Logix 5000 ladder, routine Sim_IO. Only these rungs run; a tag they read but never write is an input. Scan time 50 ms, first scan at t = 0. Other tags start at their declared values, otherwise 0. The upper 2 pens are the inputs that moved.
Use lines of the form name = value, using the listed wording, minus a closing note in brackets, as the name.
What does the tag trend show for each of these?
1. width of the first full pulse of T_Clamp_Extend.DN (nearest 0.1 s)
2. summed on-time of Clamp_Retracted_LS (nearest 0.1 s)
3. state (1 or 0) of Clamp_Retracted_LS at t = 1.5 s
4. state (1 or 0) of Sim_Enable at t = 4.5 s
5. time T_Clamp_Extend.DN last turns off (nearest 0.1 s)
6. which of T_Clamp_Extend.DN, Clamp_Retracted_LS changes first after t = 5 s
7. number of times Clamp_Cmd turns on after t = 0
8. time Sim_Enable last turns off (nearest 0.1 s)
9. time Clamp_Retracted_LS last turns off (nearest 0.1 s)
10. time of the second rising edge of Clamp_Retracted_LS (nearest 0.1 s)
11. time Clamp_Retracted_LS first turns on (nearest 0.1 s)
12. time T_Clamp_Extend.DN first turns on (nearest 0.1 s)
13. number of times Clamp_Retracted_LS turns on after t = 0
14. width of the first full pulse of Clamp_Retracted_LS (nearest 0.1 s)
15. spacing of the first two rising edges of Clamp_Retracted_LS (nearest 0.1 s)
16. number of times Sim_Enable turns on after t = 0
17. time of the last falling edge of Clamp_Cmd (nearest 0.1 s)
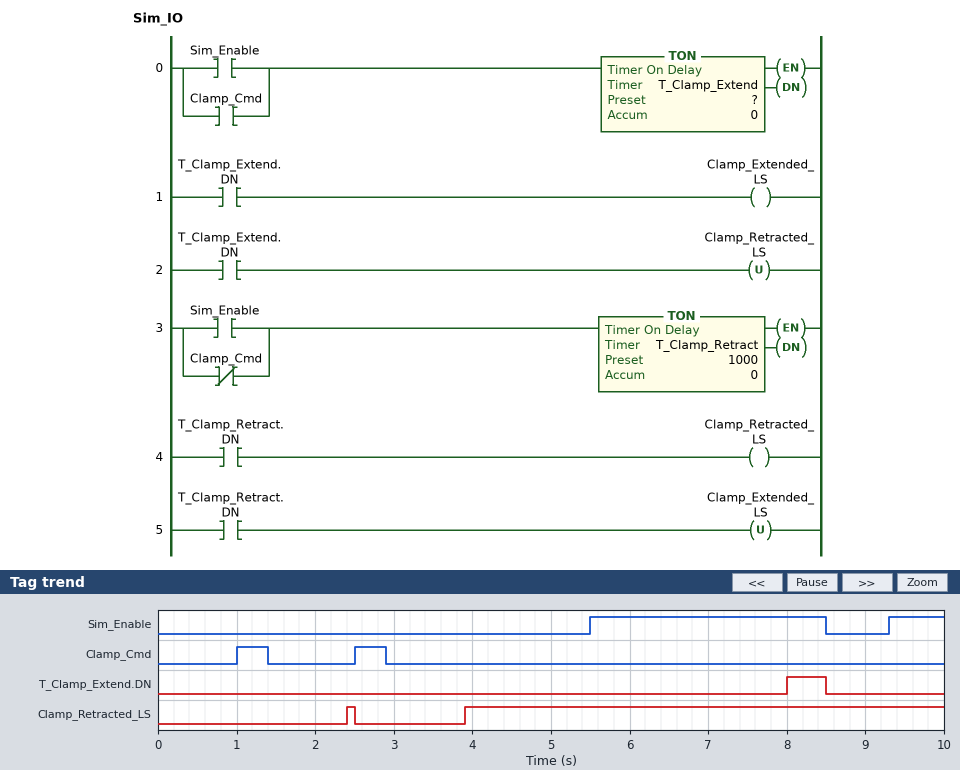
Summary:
width of the first full pulse of T_Clamp_Extend.DN = 0.5 s
summed on-time of Clamp_Retracted_LS = 6.2 s
state (1 or 0) of Clamp_Retracted_LS at t = 1.5 s = 0
state (1 or 0) of Sim_Enable at t = 4.5 s = 0
time T_Clamp_Extend.DN last turns off = 8.5 s
which of T_Clamp_Extend.DN, Clamp_Retracted_LS changes first after t = 5 s = T_Clamp_Extend.DN
number of times Clamp_Cmd turns on after t = 0 = 2
time Sim_Enable last turns off = 8.5 s
time Clamp_Retracted_LS last turns off = 2.5 s
time of the second rising edge of Clamp_Retracted_LS = 3.9 s
time Clamp_Retracted_LS first turns on = 2.4 s
time T_Clamp_Extend.DN first turns on = 8.0 s
number of times Clamp_Retracted_LS turns on after t = 0 = 2
width of the first full pulse of Clamp_Retracted_LS = 0.1 s
spacing of the first two rising edges of Clamp_Retracted_LS = 1.5 s
number of times Sim_Enable turns on after t = 0 = 2
time of the last falling edge of Clamp_Cmd = 2.9 s
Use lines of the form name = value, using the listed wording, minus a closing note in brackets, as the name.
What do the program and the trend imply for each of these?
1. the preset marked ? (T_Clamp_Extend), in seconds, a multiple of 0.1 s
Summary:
the preset marked ? (T_Clamp_Extend), in seconds, a multiple of 0.1 s = 2.5 s
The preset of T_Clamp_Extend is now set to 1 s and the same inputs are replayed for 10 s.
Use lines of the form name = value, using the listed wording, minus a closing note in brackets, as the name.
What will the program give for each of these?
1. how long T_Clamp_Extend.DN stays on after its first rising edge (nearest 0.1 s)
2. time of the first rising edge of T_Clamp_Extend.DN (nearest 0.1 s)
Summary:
how long T_Clamp_Extend.DN stays on after its first rising edge = 2.0 s
time of the first rising edge of T_Clamp_Extend.DN = 6.5 s
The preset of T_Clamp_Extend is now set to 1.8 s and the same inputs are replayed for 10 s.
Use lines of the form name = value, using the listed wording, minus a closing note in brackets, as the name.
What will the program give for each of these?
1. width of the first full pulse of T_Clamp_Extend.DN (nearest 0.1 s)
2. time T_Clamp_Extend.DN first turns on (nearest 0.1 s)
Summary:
width of the first full pulse of T_Clamp_Extend.DN = 1.2 s
time T_Clamp_Extend.DN first turns on = 7.3 s
